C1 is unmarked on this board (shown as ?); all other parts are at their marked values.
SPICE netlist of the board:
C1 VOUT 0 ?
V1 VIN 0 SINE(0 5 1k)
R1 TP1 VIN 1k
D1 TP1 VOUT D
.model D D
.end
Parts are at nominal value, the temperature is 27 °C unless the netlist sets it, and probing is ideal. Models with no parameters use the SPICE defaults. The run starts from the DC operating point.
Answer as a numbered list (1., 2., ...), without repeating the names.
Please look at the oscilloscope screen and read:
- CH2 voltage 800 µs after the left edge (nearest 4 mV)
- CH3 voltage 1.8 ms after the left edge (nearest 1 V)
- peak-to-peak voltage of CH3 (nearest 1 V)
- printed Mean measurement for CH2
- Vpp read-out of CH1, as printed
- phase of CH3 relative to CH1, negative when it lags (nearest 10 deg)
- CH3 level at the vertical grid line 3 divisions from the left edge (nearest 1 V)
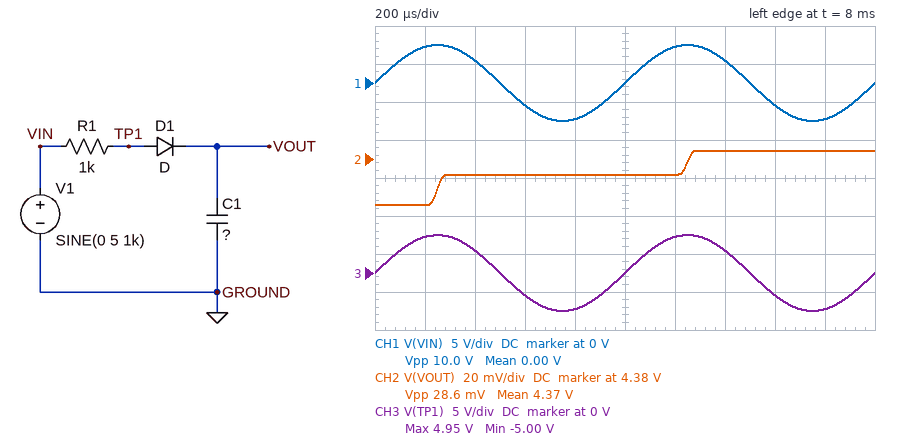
1. 4.372 V
2. -5 V
3. 10 V
4. 4.37 V
5. 10.0 V
6. 0 deg
7. -3 V
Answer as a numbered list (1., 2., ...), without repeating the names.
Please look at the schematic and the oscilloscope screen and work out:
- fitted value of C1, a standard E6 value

1. 150 nF
